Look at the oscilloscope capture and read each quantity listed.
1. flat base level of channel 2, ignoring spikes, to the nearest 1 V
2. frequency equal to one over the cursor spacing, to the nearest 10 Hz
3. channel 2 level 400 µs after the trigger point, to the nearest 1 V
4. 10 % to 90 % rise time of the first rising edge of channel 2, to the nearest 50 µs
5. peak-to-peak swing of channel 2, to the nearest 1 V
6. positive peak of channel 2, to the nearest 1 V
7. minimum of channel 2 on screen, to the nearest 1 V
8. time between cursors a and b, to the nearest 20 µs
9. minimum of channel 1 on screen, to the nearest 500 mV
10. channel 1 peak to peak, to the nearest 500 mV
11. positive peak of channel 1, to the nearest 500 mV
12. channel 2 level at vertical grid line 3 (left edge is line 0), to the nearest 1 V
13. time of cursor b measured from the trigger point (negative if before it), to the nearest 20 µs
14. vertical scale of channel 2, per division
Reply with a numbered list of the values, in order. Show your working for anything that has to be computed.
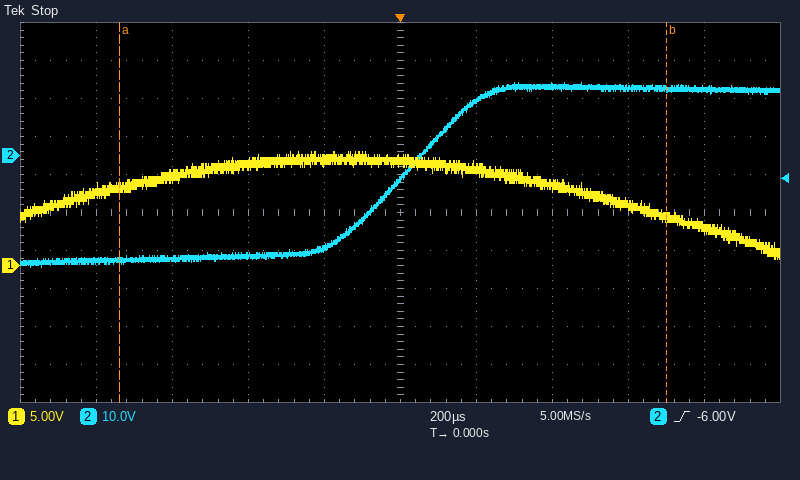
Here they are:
1. -27 V
2. 1 / 1.44 ms ≈ 690 Hz
3. 18 V
4. 350 µs
5. 19 V − (-29 V) = 48 V
6. 19 V
7. -29 V
8. 1.44 ms
9. 1.0 V
10. 15.0 V − (1.0 V) = 14.0 V
11. 15.0 V
12. -26 V
13. +700 µs
14. 10 V
